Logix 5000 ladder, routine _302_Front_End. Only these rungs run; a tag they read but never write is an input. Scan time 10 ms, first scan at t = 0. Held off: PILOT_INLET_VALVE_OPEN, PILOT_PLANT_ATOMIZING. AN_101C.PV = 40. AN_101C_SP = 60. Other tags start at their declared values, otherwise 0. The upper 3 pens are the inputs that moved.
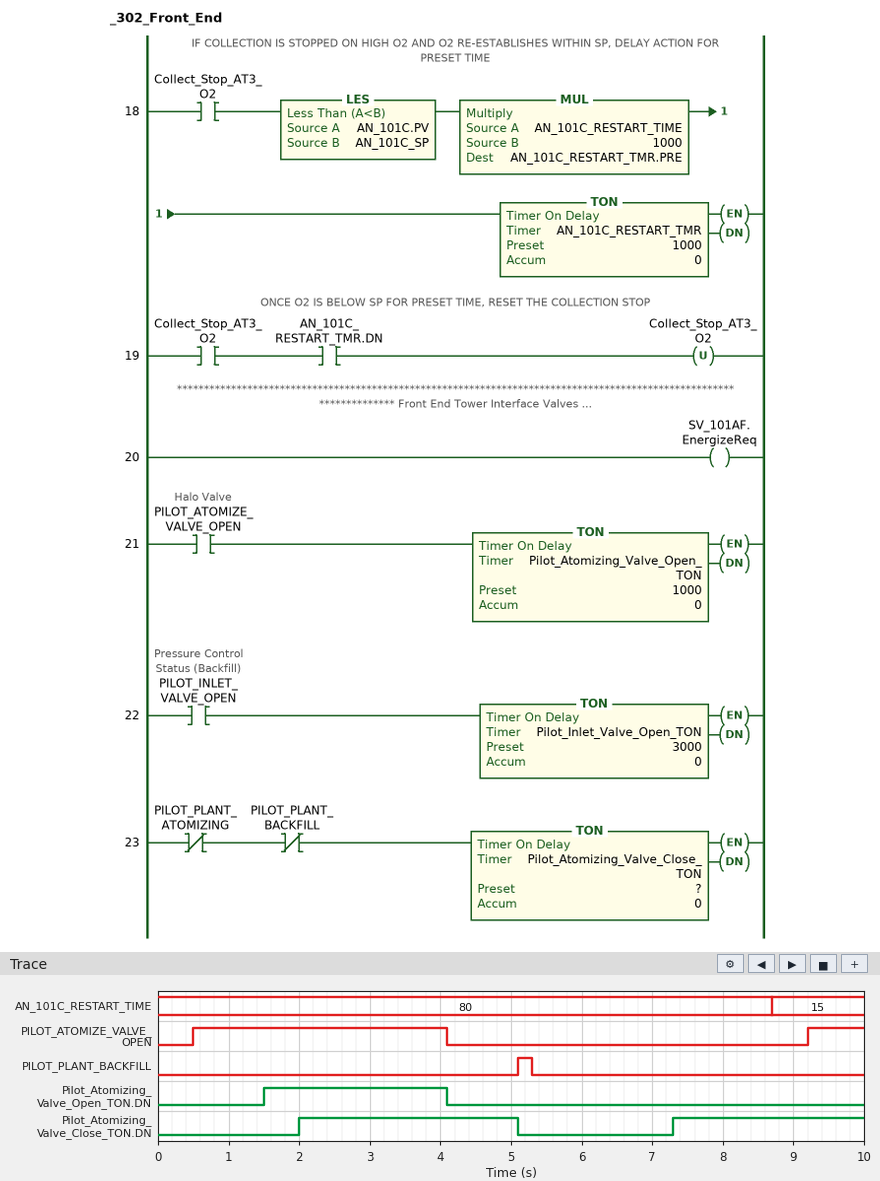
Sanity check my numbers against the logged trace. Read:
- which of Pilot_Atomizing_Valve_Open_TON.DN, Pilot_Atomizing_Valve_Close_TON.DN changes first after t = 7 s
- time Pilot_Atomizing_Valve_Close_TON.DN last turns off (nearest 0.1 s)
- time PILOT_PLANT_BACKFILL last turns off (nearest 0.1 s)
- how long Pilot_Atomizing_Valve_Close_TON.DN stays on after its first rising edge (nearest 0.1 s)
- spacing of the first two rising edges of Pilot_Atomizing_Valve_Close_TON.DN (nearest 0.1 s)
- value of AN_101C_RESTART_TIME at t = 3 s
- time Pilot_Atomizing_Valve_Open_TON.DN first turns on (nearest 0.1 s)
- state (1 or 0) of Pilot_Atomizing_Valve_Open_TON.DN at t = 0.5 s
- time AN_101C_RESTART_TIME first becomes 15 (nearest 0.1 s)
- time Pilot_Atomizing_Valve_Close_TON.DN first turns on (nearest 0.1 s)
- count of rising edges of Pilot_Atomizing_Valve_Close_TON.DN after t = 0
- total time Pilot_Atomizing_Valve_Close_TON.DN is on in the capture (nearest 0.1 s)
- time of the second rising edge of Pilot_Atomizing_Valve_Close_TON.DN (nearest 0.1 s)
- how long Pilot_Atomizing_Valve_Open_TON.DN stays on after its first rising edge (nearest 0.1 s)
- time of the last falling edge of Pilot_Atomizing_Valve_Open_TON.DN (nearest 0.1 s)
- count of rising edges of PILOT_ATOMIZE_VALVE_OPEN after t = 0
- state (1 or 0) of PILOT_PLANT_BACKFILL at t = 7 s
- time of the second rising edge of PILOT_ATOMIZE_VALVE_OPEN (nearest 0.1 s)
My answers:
Pilot_Atomizing_Valve_Close_TON.DN
5.1 s
5.3 s
3.1 s
5.3 s
80
1.5 s
0
8.7 s
2.0 s
2
5.8 s
7.3 s
2.6 s
4.1 s
2
0
9.2 s
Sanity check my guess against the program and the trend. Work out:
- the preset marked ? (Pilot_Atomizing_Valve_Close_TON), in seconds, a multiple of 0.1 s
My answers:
2.0 s
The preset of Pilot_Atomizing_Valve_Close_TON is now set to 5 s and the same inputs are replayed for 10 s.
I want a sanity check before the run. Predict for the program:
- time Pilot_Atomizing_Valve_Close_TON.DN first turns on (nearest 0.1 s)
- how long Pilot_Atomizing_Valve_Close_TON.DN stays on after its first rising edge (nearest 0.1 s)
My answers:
5.0 s
0.1 s
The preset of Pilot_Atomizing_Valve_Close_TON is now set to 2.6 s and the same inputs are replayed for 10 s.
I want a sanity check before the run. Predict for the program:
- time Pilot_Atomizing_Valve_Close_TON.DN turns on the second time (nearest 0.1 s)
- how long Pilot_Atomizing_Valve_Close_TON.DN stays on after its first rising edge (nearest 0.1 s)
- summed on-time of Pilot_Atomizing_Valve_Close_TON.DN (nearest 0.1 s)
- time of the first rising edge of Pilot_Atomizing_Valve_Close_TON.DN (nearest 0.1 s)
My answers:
7.9 s
2.5 s
4.6 s
2.6 s
